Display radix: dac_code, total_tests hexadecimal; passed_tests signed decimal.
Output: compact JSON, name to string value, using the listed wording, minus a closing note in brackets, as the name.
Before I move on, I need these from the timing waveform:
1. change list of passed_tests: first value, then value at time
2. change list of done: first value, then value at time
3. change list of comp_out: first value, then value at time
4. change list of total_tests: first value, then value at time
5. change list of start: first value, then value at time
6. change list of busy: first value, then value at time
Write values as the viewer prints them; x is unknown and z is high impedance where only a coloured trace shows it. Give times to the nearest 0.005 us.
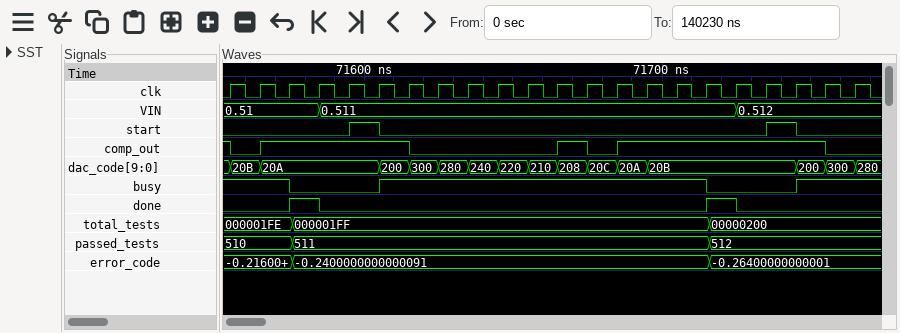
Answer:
{"change list of passed_tests: first value, then value at time": "510, 511 at 71.575 us, 512 at 71.715 us", "change list of done: first value, then value at time": "0, 1 at 71.575 us, 0 at 71.585 us, 1 at 71.715 us, 0 at 71.725 us", "change list of comp_out: first value, then value at time": "1, 0 at 71.555 us, 1 at 71.565 us, 0 at 71.615 us, 1 at 71.665 us, 0 at 71.675 us, 1 at 71.685 us, 0 at 71.755 us", "change list of total_tests: first value, then value at time": "000001FE, 000001FF at 71.575 us, 00000200 at 71.715 us", "change list of start: first value, then value at time": "0, 1 at 71.595 us, 0 at 71.605 us, 1 at 71.735 us, 0 at 71.745 us", "change list of busy: first value, then value at time": "1, 0 at 71.575 us, 1 at 71.605 us, 0 at 71.715 us, 1 at 71.745 us"}
